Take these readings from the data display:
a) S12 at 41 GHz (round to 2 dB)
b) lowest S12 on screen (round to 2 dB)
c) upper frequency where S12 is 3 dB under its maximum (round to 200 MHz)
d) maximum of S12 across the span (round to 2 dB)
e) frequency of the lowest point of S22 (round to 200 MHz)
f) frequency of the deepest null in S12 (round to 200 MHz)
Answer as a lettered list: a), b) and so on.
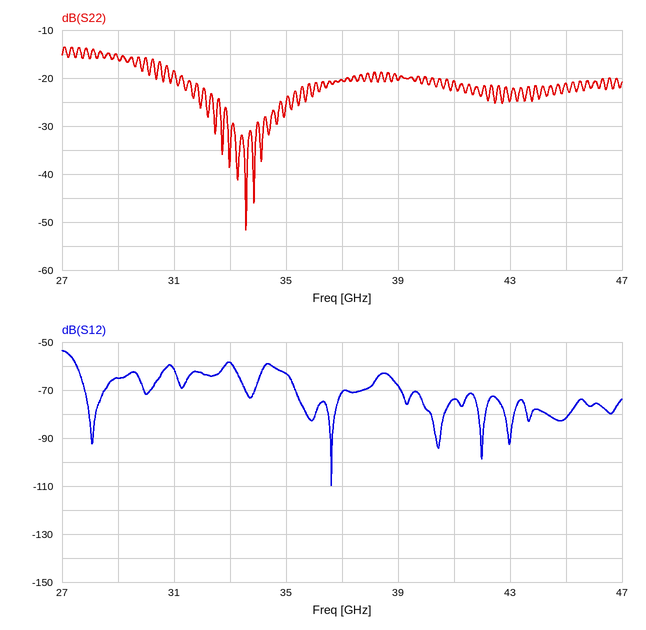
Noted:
a) -74 dB
b) -110 dB
c) 27.4 GHz
d) -54 dB
e) 33.6 GHz
f) 36.6 GHz
